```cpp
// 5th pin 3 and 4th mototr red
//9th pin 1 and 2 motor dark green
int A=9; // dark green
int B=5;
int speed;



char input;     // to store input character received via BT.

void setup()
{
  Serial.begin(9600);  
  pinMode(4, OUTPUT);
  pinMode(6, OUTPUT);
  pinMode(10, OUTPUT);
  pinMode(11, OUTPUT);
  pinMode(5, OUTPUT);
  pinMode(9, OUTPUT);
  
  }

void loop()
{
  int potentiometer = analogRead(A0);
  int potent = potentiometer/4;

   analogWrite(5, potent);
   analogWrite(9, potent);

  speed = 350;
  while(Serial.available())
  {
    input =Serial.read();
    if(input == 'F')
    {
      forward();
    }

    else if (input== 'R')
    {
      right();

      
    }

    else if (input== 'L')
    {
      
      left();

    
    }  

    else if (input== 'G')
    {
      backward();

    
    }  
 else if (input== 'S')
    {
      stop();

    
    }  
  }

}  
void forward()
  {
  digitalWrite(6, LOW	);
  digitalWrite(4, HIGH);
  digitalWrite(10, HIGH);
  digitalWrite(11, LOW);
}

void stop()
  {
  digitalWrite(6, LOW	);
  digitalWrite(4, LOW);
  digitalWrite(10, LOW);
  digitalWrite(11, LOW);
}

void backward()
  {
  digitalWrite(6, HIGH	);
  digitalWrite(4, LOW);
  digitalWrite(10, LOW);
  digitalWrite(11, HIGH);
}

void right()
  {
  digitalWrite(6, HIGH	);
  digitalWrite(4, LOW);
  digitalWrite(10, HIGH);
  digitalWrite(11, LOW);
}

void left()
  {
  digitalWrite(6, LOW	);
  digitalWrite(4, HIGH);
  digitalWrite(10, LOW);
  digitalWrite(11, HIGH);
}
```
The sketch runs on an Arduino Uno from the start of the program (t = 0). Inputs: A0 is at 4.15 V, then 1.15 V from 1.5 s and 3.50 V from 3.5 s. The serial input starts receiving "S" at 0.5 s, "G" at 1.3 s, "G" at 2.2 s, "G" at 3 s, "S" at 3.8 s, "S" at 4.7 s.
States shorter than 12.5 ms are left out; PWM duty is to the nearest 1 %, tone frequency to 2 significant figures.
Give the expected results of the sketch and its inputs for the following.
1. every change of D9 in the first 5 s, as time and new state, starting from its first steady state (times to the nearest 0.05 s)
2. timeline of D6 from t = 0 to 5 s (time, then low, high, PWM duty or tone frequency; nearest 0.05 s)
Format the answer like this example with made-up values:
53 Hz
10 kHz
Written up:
0 s PWM 83 %; 1.5 s PWM 23 %; 3.5 s PWM 70 %
0 s low; 1.3 s high; 3.8 s low
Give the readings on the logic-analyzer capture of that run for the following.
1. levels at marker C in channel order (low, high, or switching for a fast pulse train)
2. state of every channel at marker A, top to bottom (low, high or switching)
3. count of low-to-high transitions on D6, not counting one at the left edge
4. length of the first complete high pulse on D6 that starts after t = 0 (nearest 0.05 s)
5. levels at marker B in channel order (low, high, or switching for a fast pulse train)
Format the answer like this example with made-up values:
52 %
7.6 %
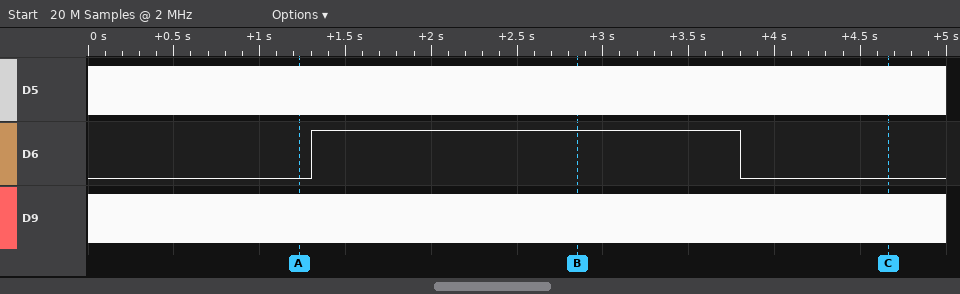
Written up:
D5 switching, D6 low, D9 switching
D5 switching, D6 low, D9 switching
1
2.50 s
D5 switching, D6 high, D9 switching
